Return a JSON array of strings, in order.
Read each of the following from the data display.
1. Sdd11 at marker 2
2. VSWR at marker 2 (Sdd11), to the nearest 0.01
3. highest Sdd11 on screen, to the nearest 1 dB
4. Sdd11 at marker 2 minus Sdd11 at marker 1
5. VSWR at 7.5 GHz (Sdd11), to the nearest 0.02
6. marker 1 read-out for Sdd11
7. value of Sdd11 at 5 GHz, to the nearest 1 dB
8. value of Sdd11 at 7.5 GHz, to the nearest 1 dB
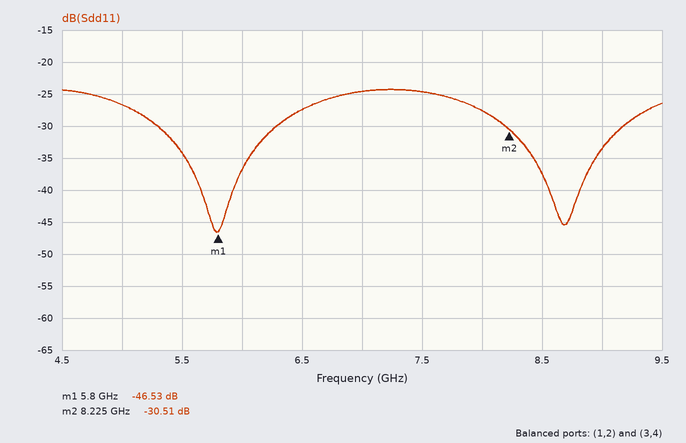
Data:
["-30.51 dB", "1.06", "-24 dB", "16.02 dB", "1.12", "-46.53 dB", "-27 dB", "-25 dB"]
